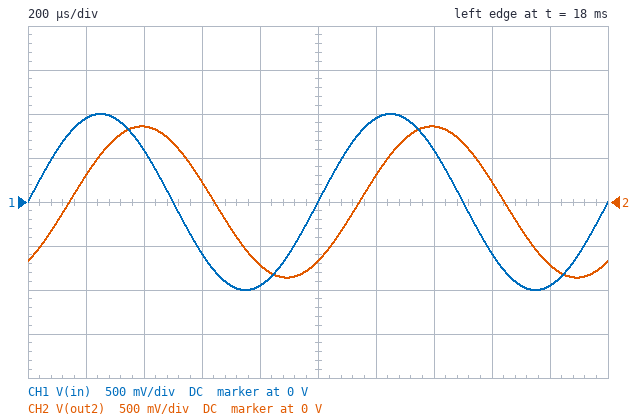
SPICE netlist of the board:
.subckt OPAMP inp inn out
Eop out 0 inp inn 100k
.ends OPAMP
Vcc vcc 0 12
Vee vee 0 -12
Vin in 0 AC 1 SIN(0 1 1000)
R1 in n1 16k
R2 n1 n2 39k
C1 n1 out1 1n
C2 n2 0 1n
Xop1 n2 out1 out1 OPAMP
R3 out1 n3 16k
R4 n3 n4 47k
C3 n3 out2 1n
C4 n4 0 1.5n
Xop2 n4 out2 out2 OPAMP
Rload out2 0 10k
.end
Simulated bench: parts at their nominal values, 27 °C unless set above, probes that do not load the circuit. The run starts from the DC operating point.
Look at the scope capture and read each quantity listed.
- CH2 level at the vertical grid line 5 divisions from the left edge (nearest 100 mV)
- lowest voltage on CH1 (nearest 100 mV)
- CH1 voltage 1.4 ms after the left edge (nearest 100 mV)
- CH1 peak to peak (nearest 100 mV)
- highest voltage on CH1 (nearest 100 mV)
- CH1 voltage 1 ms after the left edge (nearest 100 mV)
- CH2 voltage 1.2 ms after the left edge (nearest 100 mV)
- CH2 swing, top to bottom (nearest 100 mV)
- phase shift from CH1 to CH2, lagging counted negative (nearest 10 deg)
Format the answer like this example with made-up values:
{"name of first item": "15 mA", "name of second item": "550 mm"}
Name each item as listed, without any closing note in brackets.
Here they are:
{"CH2 level at the vertical grid line 5 divisions from the left edge": "-700 mV", "lowest voltage on CH1": "-1.0 V", "CH1 voltage 1.4 ms after the left edge": "600 mV", "CH1 peak to peak": "2.0 V", "highest voltage on CH1": "1.0 V", "CH1 voltage 1 ms after the left edge": "0 V", "CH2 voltage 1.2 ms after the left edge": "300 mV", "CH2 swing, top to bottom": "1.7 V", "phase shift from CH1 to CH2, lagging counted negative": "-50 deg"}
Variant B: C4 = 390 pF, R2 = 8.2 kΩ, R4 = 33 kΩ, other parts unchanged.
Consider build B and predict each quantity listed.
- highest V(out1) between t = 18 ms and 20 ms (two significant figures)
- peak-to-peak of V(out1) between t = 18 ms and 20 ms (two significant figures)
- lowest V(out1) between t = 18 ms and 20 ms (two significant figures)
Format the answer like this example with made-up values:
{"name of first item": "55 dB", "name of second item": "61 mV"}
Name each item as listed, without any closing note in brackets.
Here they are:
{"highest V(out1) between t = 18 ms and 20 ms": "990 mV", "peak-to-peak of V(out1) between t = 18 ms and 20 ms": "2.0 V", "lowest V(out1) between t = 18 ms and 20 ms": "-990 mV"}
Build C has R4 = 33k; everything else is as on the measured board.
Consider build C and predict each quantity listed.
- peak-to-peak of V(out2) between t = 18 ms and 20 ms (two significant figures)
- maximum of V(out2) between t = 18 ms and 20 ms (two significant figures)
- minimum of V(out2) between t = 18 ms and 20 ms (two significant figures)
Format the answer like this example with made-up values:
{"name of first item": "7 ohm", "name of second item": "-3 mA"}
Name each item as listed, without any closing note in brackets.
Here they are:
{"peak-to-peak of V(out2) between t = 18 ms and 20 ms": "1.8 V", "maximum of V(out2) between t = 18 ms and 20 ms": "900 mV", "minimum of V(out2) between t = 18 ms and 20 ms": "-900 mV"}
